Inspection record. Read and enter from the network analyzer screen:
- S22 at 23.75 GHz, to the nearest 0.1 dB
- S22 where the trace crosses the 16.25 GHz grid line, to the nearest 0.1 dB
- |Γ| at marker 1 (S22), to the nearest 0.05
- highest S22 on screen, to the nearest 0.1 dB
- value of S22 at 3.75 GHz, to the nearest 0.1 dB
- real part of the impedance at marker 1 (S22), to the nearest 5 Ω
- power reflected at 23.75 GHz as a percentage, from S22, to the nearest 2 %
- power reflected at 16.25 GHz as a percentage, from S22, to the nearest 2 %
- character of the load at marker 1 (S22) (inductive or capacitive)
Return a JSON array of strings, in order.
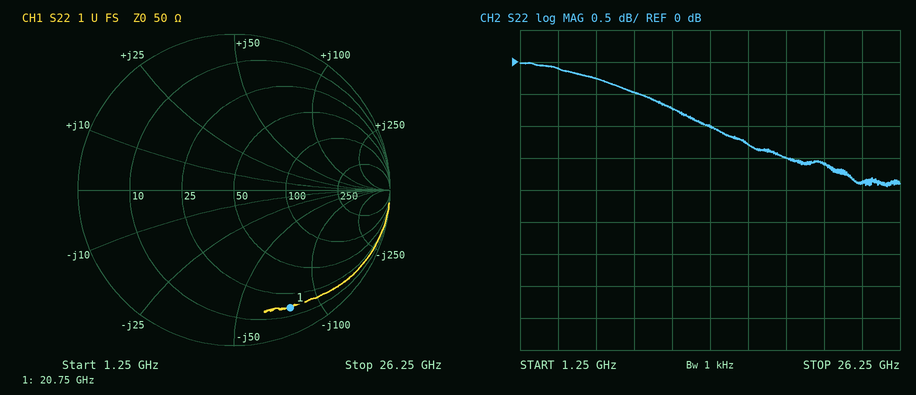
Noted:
["-1.9 dB", "-1.3 dB", "0.85", "0.0 dB", "-0.1 dB", "15 Ω", "64 %", "74 %", "capacitive"]
